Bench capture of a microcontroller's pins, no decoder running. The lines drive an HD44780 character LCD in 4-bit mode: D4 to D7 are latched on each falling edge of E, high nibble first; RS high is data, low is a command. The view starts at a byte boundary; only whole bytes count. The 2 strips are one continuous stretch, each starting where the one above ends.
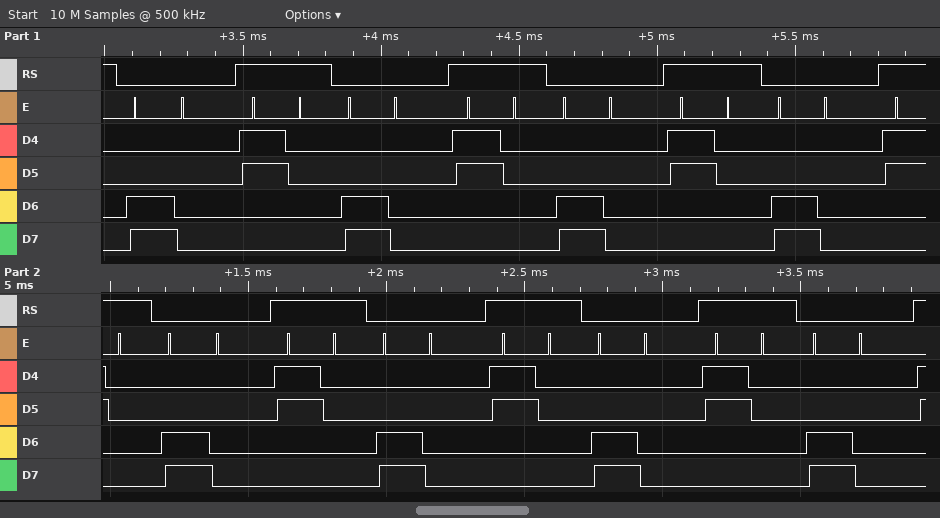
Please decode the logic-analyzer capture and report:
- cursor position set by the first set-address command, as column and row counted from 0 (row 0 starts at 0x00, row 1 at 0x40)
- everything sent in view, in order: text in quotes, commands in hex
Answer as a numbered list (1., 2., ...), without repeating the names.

1. column 0, row 1
2. 0xC0 "0" 0xC0 "0" 0xC0 "0" 0xC0 "0" 0xC0 "0" 0xC0 "0" 0xC0 "0" 0xC0
